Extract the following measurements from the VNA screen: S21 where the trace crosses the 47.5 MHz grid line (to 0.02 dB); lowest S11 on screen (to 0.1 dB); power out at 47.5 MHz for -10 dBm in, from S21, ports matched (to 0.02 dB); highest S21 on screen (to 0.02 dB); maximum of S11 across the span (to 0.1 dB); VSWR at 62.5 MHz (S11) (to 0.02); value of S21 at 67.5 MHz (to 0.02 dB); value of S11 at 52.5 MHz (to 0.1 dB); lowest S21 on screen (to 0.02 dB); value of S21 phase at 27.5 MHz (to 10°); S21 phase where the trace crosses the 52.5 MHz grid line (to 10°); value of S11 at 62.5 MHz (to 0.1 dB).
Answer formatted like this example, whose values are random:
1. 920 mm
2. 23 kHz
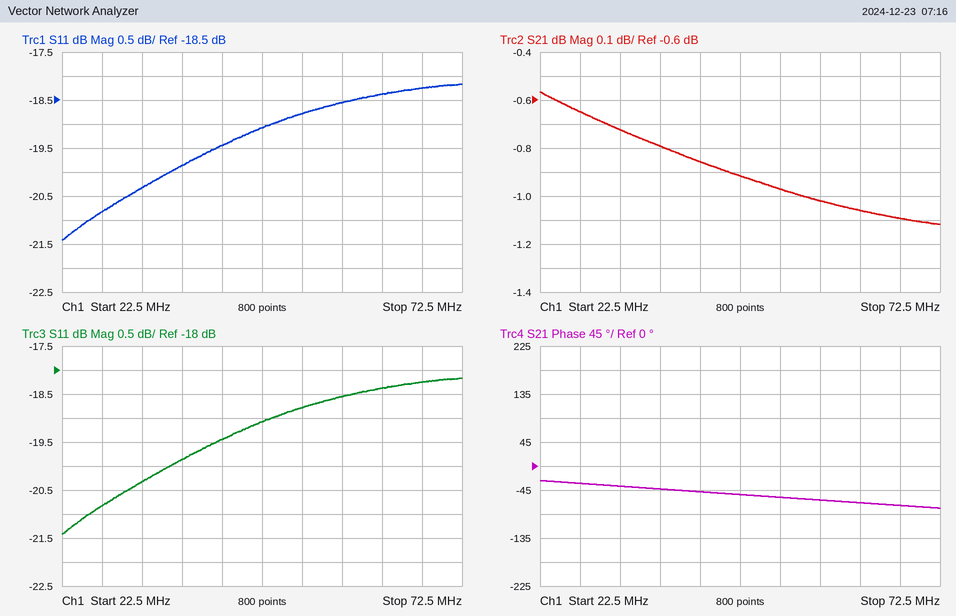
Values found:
1. -0.92 dB
2. -21.4 dB
3. -10.92 dBm
4. -0.56 dB
5. -18.2 dB
6. 1.28
7. -1.10 dB
8. -18.8 dB
9. -1.12 dB
10. -30°
11. -60°
12. -18.4 dB
